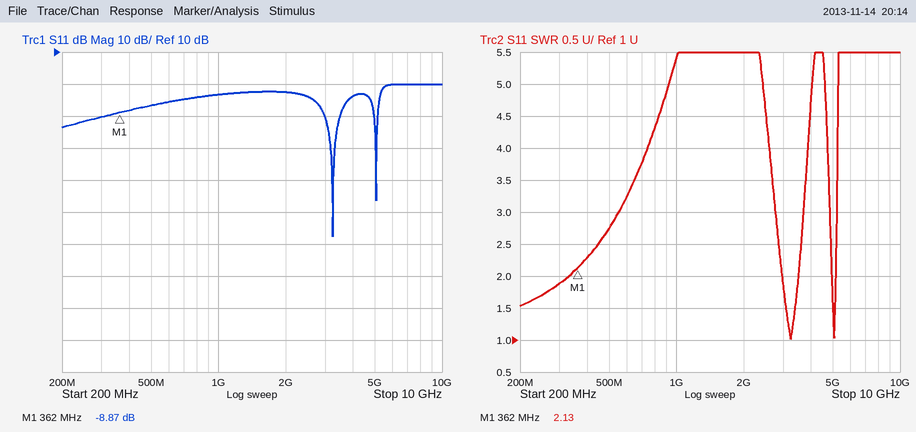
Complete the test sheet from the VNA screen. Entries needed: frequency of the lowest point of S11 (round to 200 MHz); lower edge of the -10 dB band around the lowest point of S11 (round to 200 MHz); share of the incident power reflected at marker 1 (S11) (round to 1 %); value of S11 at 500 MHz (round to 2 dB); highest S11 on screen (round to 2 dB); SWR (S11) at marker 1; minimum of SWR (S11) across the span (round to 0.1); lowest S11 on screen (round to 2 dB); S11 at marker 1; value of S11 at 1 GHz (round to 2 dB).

3.2 GHz
3.0 GHz
13 %
-6 dB
0 dB
2.13
1.0
-48 dB
-8.87 dB
-4 dB
